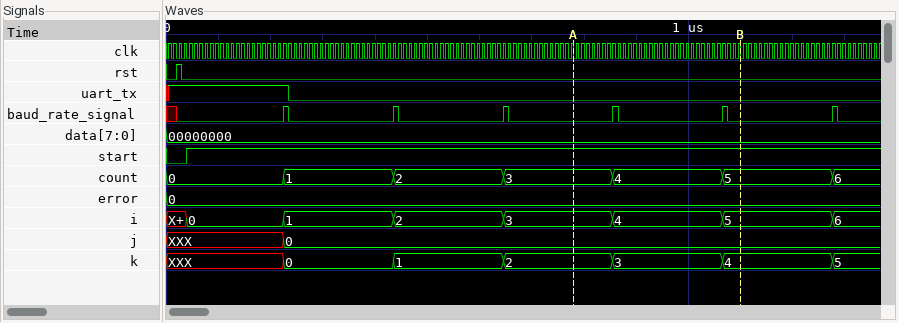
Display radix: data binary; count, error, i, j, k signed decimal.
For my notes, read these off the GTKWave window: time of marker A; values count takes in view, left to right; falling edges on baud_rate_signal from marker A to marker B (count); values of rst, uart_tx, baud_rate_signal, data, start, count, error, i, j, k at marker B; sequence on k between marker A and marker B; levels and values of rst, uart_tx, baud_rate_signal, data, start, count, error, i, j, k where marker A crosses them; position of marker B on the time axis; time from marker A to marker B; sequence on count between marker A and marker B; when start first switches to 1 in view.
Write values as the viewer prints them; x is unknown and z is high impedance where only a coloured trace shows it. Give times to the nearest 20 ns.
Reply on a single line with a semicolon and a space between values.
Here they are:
780 ns; 0, 1, 2, 3, 4, 5, 6; 2; rst=0, uart_tx=0, baud_rate_signal=0, data=00000000, start=1, count=5, error=0, i=5, j=0, k=4; 2, 3, 4; rst=0, uart_tx=0, baud_rate_signal=0, data=00000000, start=1, count=3, error=0, i=3, j=0, k=2; 1100 ns; 320 ns; 3, 4, 5; 40 ns
